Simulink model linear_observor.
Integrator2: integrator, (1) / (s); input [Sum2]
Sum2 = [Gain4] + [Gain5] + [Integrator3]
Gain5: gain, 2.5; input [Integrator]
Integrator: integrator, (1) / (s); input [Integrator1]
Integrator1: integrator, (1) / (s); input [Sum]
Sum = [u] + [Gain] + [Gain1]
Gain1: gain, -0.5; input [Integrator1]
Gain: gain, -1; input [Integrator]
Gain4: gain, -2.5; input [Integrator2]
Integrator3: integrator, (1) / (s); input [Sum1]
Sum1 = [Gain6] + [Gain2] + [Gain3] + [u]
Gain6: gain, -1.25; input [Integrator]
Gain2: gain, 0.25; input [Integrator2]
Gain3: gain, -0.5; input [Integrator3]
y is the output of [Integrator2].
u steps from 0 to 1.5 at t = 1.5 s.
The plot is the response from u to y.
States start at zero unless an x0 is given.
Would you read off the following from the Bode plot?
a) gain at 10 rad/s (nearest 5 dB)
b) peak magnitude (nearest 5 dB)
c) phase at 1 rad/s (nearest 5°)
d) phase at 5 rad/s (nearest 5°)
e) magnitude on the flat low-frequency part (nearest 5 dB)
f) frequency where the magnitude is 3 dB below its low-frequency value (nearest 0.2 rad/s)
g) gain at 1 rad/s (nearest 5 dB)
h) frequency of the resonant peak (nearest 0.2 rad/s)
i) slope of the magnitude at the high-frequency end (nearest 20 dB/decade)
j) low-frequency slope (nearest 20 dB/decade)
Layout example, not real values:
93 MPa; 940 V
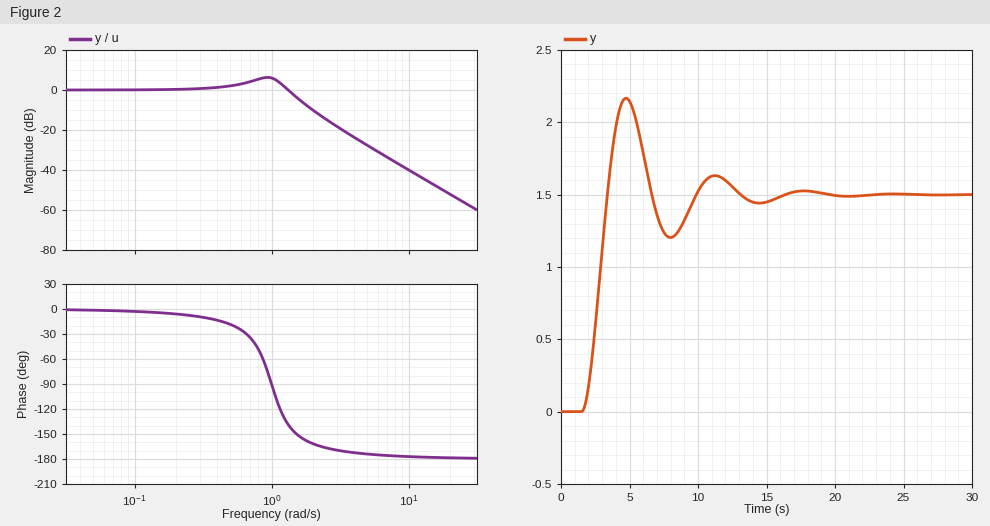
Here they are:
-40 dB; 5 dB; -90°; -175°; 0 dB; 1.4 rad/s; 5 dB; 1.0 rad/s; -40 dB/decade; 0 dB/decade
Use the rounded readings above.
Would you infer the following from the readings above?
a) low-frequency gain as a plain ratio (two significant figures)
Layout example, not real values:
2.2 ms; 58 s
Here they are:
1.0
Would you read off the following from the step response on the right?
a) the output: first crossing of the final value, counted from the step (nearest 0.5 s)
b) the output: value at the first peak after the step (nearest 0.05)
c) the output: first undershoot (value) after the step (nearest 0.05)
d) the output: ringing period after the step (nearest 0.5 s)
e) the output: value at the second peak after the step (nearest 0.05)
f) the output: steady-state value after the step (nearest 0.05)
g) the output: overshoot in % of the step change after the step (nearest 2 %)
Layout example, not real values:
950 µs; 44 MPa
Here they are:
2.0 s; 2.15; 1.20; 6.5 s; 1.65; 1.50; 44 %
